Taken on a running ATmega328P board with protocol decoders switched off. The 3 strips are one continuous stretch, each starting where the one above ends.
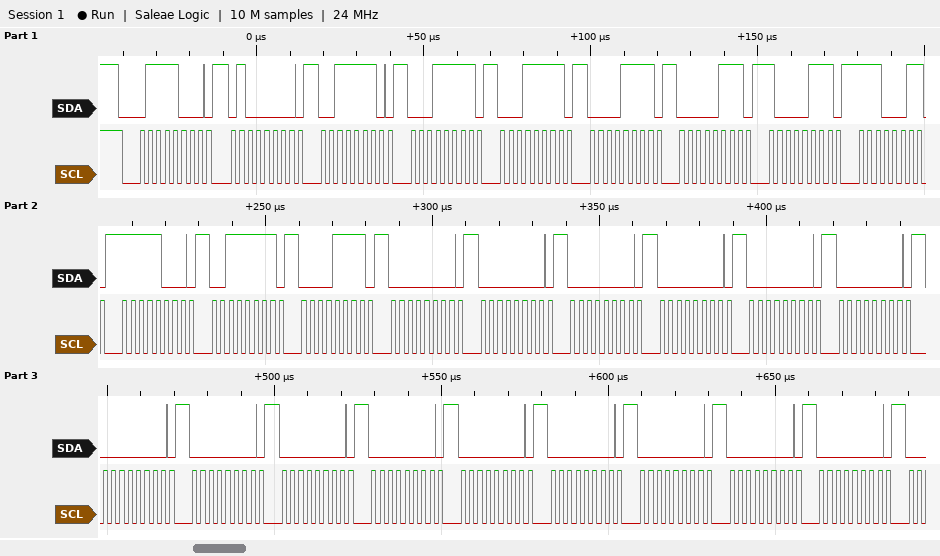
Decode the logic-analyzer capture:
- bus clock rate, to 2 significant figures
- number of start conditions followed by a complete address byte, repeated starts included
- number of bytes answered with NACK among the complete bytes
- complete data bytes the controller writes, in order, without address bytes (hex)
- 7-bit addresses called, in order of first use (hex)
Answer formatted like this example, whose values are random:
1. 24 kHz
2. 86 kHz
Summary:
1. 400 kHz
2. 1
3. 0
4. 40 3E 1F 1F 0F 07 87 E3 F8 3F 0F 00 00 00 00 00 00 00 00 00 00 00 00 00 00 00
5. 0x3C
